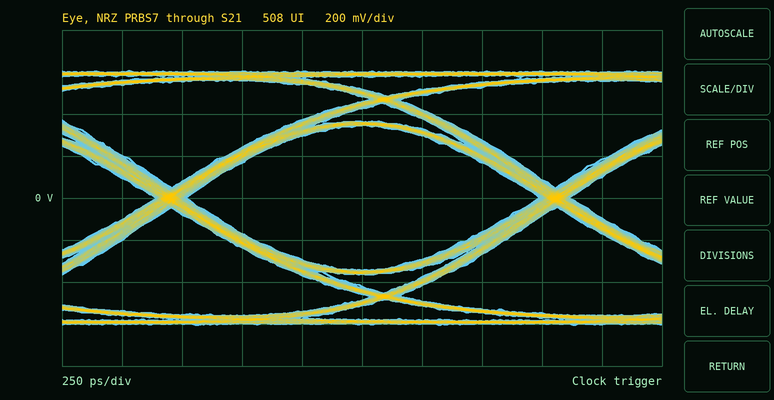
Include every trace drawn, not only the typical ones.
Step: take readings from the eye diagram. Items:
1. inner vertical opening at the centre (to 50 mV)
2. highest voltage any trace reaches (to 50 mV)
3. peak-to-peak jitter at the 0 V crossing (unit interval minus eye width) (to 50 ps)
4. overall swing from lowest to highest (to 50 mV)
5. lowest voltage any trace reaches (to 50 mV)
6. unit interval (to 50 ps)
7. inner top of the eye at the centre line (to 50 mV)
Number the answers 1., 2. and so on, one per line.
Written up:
1. 700 mV
2. 600 mV
3. 150 ps
4. 1.20 V
5. -600 mV
6. 1.60 ns
7. 350 mV
